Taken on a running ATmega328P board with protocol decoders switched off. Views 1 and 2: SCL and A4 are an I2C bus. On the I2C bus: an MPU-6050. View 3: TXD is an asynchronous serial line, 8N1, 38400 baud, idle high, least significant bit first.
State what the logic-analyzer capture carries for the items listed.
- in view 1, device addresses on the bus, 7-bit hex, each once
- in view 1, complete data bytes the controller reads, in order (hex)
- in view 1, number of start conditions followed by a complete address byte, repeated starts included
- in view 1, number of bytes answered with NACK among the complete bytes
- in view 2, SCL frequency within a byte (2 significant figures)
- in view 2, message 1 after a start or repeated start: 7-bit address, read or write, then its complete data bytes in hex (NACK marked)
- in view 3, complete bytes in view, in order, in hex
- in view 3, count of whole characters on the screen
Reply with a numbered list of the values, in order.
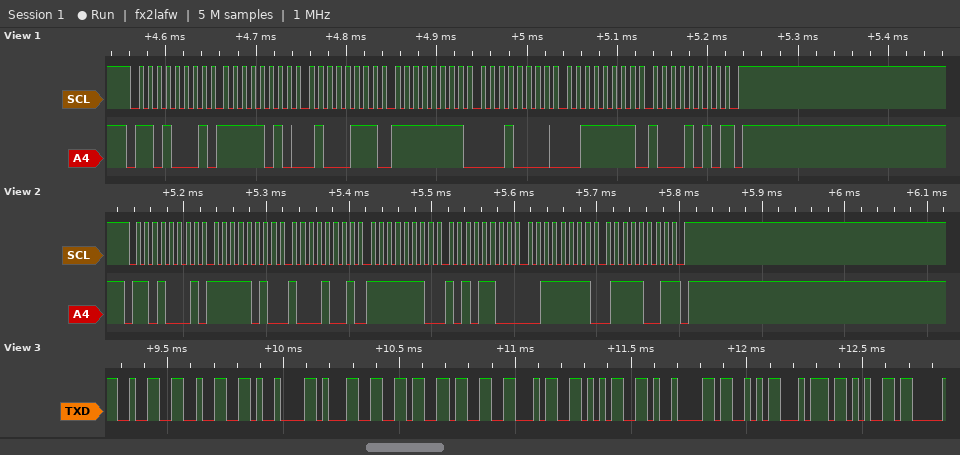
1. 0x68
2. FA 47 FF 10 3F 8A
3. 1
4. 1
5. 100 kHz
6. 0x68 read: FA 89 FE AC 3F 79 NACK
7. 32 32 09 31 36 33 34 35 09 53 74 65
8. 12
